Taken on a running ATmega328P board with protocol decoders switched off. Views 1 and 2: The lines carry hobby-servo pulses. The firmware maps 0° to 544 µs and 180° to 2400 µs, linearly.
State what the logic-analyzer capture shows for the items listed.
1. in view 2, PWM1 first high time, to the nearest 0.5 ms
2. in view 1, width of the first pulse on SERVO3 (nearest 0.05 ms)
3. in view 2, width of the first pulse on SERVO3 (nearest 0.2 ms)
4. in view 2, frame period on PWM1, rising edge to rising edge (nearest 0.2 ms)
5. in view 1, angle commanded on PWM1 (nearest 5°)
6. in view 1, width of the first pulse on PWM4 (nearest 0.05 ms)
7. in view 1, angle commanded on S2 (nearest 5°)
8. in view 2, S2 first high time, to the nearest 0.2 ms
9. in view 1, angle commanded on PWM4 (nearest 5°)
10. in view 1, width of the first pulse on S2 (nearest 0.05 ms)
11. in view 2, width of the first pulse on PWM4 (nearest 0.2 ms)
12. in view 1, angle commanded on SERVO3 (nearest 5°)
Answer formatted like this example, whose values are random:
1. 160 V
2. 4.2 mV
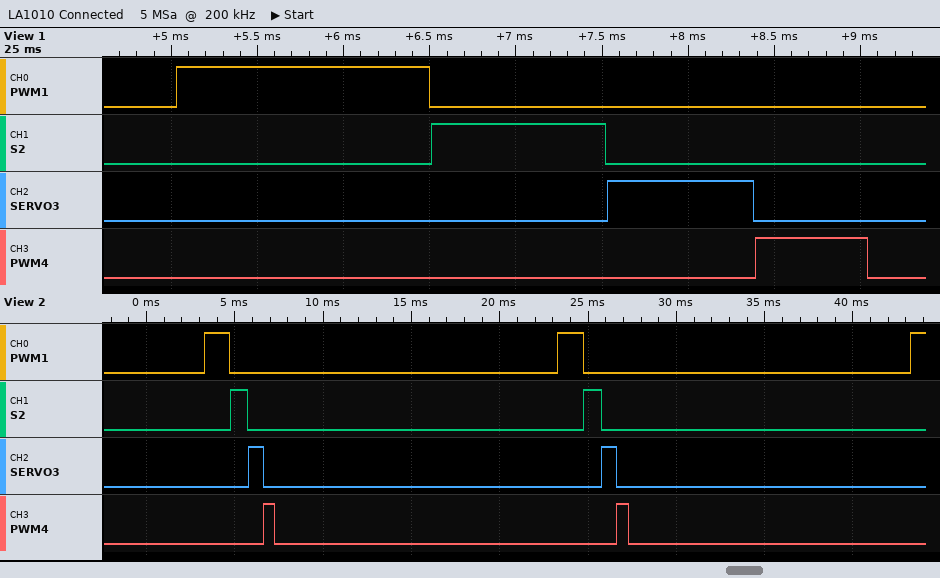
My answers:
1. 1.5 ms
2. 0.85 ms
3. 0.8 ms
4. 20.0 ms
5. 90°
6. 0.65 ms
7. 45°
8. 1.0 ms
9. 10°
10. 1.00 ms
11. 0.6 ms
12. 30°
